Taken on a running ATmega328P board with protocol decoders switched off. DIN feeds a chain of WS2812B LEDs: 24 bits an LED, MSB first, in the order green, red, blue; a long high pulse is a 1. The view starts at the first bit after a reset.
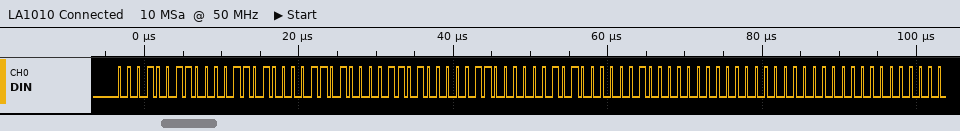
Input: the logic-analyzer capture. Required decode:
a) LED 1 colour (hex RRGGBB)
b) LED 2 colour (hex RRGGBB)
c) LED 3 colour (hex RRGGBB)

#0D130D
#060D05
#000200
